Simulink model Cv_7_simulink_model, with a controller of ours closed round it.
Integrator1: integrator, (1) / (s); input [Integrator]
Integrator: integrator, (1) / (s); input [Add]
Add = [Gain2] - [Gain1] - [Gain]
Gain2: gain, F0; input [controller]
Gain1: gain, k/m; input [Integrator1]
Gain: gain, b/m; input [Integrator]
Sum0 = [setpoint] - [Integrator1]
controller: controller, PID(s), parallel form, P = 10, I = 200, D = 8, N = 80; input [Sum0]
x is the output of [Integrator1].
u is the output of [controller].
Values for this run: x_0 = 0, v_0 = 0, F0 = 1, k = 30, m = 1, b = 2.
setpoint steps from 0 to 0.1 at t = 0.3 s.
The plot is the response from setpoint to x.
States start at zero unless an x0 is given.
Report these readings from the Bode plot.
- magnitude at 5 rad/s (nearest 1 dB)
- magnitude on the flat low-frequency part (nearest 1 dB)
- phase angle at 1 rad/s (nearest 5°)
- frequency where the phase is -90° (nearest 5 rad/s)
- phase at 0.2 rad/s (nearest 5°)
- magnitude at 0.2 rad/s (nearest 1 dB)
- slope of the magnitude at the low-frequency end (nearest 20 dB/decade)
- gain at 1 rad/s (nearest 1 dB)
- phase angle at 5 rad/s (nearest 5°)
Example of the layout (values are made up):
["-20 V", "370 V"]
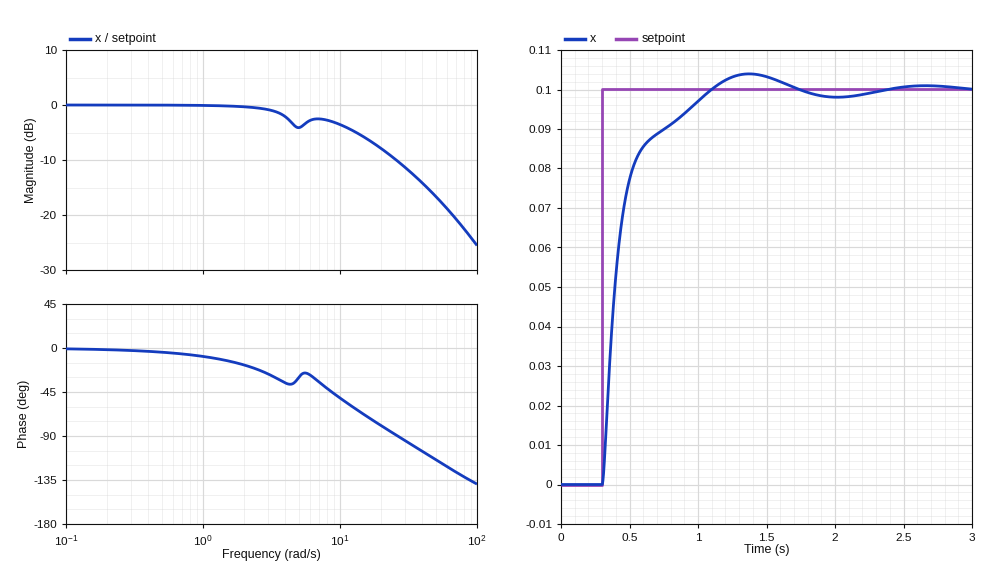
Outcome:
["-4 dB", "0 dB", "-10°", "25 rad/s", "0°", "0 dB", "0 dB/decade", "0 dB", "-30°"]
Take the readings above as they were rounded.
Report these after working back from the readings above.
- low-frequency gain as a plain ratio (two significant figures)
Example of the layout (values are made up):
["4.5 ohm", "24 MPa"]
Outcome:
["1.0"]
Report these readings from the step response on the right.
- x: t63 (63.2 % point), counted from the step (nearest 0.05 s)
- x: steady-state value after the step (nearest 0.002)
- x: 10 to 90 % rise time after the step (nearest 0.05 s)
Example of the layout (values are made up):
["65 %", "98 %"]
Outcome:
["0.15 s", "0.100", "0.45 s"]
